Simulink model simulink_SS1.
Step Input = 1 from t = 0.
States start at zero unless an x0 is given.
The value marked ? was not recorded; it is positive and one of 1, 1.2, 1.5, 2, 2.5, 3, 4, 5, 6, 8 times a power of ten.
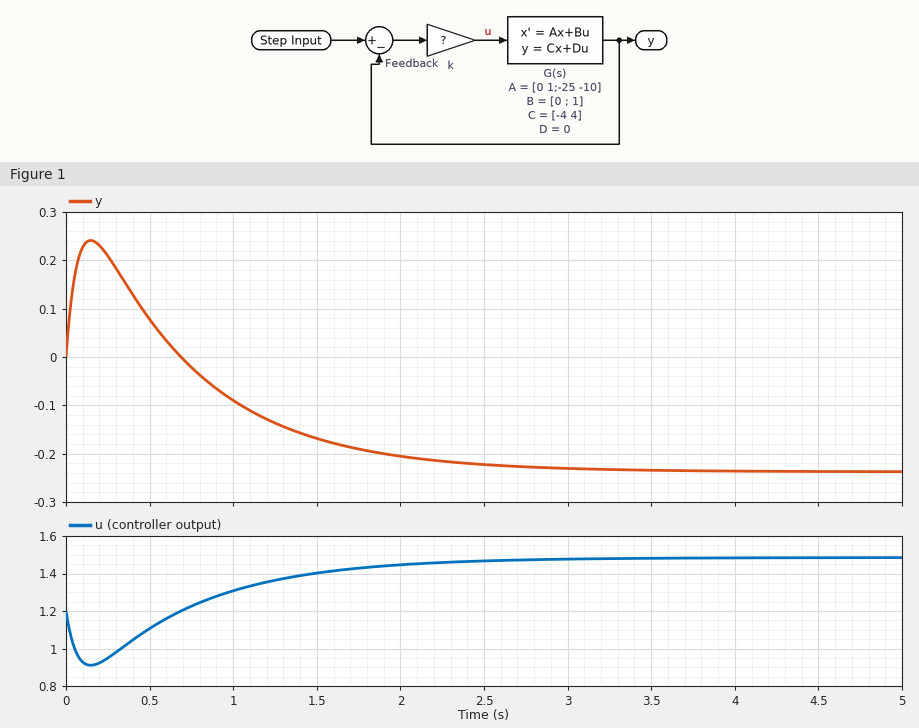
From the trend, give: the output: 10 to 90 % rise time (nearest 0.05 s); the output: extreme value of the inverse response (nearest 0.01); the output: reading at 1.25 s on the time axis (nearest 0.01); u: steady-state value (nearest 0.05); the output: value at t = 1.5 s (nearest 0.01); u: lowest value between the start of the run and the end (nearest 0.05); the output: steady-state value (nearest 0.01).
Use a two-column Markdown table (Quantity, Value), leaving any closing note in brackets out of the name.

| Quantity | Value |
|---|---|
| the output: 10 to 90 % rise time | 1.45 s |
| the output: extreme value of the inverse response | 0.24 |
| the output: reading at 1.25 s on the time axis | -0.14 |
| u: steady-state value | 1.50 |
| the output: value at t = 1.5 s | -0.17 |
| u: lowest value between the start of the run and the end | 0.90 |
| the output: steady-state value | -0.24 |
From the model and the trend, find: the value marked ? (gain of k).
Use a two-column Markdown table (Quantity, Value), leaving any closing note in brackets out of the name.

| Quantity | Value |
|---|---|
| the value marked ? | 1.2 |
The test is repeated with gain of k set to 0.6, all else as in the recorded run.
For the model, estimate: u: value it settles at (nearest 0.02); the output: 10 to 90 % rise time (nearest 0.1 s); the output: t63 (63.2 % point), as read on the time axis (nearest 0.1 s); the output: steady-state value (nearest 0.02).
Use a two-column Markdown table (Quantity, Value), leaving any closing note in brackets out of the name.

| Quantity | Value |
|---|---|
| u: value it settles at | 0.66 |
| the output: 10 to 90 % rise time | 1.0 s |
| the output: t63 (63.2 % point), as read on the time axis | 1.1 s |
| the output: steady-state value | -0.10 |
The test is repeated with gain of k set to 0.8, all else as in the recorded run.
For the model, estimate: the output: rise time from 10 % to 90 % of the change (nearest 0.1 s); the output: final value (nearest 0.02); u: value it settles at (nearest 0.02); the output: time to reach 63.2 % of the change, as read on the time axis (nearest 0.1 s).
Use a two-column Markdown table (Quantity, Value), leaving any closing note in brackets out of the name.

| Quantity | Value |
|---|---|
| the output: rise time from 10 % to 90 % of the change | 1.1 s |
| the output: final value | -0.14 |
| u: value it settles at | 0.92 |
| the output: time to reach 63.2 % of the change, as read on the time axis | 1.2 s |
